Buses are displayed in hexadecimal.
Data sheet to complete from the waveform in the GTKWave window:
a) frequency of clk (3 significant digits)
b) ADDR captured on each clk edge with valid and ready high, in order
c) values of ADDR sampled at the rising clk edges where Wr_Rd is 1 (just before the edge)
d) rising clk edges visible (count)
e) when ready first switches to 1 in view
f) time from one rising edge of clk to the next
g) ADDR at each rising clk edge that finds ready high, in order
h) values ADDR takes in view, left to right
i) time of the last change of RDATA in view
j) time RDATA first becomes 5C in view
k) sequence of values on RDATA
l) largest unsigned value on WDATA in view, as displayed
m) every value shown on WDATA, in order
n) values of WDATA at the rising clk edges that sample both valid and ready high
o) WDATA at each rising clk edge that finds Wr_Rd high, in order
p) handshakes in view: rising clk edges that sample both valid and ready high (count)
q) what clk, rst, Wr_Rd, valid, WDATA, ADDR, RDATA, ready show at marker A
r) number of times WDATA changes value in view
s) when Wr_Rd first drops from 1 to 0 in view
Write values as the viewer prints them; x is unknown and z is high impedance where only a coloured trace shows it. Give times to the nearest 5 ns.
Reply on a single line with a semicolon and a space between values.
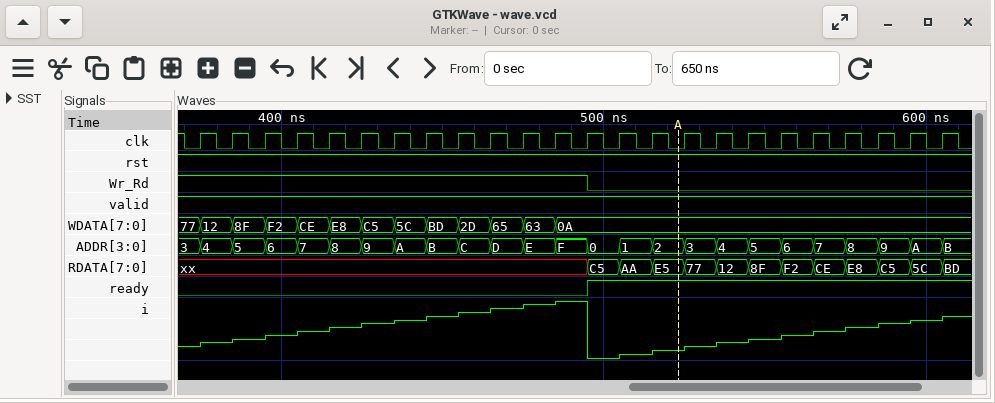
100 MHz; 0, 1, 2, 3, 4, 5, 6, 7, 8, 9, A; 3, 4, 5, 6, 7, 8, 9, A, B, C, D, E, F; 24; 495 ns; 10 ns; 0, 1, 2, 3, 4, 5, 6, 7, 8, 9, A; 3, 4, 5, 6, 7, 8, 9, A, B, C, D, E, F, 0, 1, 2, 3, 4, 5, 6, 7, 8, 9, A, B; 605 ns; 595 ns; xx, C5, AA, E5, 77, 12, 8F, F2, CE, E8, C5, 5C, BD; F2; 77, 12, 8F, F2, CE, E8, C5, 5C, BD, 2D, 65, 63, 0A; 0A, 0A, 0A, 0A, 0A, 0A, 0A, 0A, 0A, 0A, 0A; 77, 12, 8F, F2, CE, E8, C5, 5C, BD, 2D, 65, 63, 0A; 11; clk=0, rst=1, Wr_Rd=0, valid=1, WDATA=0A, ADDR=2, RDATA=E5, ready=1; 12; 495 ns
